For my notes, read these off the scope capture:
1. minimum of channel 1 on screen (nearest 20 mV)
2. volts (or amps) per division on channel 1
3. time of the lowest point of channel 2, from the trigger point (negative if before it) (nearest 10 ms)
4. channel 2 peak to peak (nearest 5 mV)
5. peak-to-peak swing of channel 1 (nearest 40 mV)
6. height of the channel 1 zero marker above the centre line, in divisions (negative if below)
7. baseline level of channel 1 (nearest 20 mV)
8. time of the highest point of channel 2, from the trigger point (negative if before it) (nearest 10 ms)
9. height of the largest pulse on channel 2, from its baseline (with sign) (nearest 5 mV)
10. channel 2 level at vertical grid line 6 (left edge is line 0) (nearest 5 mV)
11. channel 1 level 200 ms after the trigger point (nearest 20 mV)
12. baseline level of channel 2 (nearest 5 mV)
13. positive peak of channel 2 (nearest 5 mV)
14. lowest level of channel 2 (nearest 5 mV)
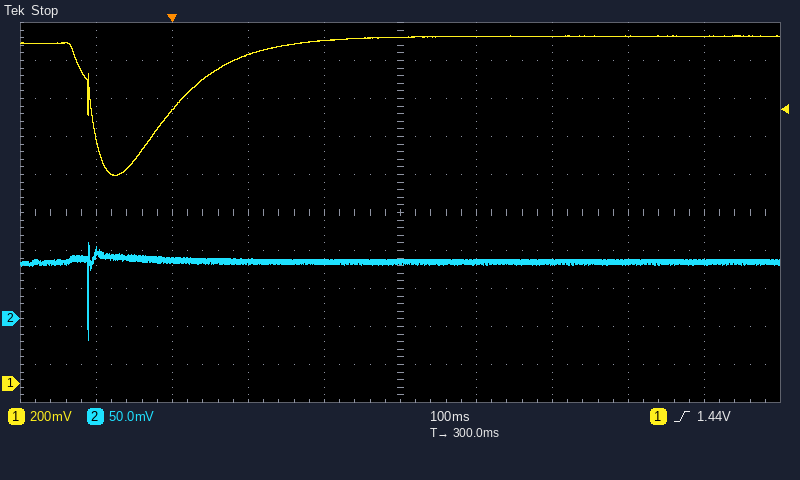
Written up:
1.10 V
200 mV
-110 ms
130 mV
720 mV
-4.5 div
1.82 V
-110 ms
-105 mV
75 mV
1.80 V
75 mV
100 mV
-30 mV
